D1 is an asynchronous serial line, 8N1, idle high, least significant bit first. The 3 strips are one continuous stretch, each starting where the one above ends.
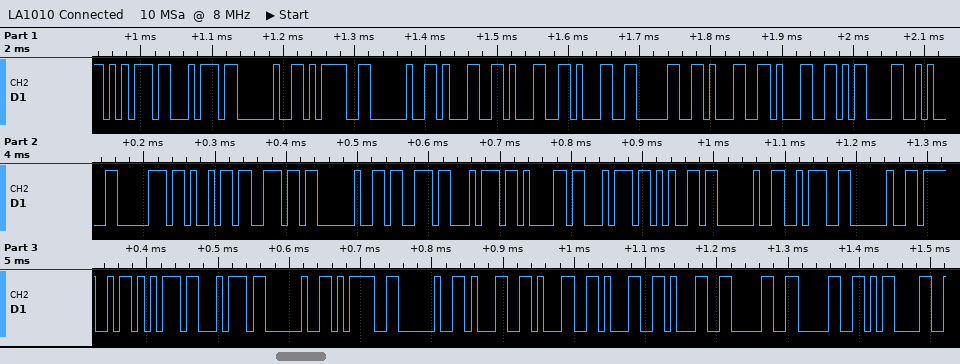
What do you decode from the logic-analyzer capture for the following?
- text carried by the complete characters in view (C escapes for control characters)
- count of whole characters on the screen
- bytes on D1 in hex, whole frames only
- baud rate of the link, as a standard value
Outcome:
"ut = 111011\r\npin state : Out = 111100\r"
38
0x75 0x74 0x20 0x3D 0x20 0x31 0x31 0x31 0x30 0x31 0x31 0x0D 0x0A 0x70 0x69 0x6E 0x20 0x73 0x74 0x61 0x74 0x65 0x20 0x3A 0x20 0x4F 0x75 0x74 0x20 0x3D 0x20 0x31 0x31 0x31 0x31 0x30 0x30 0x0D
115200 baud
